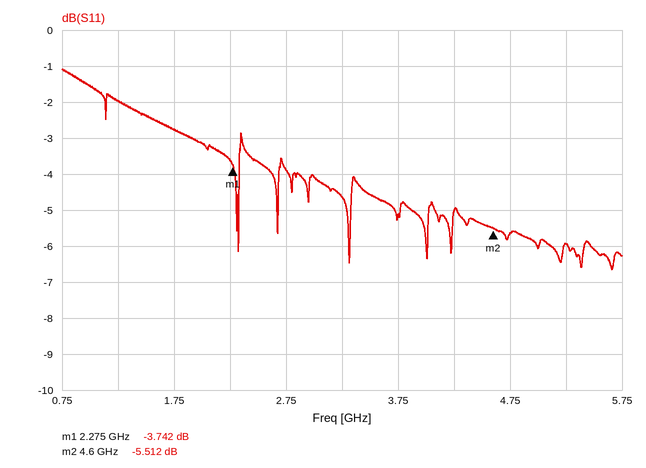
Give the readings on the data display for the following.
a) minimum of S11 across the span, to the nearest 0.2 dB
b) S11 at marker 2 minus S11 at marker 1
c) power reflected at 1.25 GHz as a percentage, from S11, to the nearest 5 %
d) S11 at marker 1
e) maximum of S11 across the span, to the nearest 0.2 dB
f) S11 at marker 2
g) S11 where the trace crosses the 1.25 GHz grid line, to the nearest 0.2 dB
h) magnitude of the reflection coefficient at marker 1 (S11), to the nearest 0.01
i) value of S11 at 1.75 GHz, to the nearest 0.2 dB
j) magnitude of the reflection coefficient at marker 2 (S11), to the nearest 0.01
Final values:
-6.6 dB
-1.770 dB
65 %
-3.742 dB
-1.0 dB
-5.512 dB
-2.0 dB
0.65
-2.8 dB
0.53
